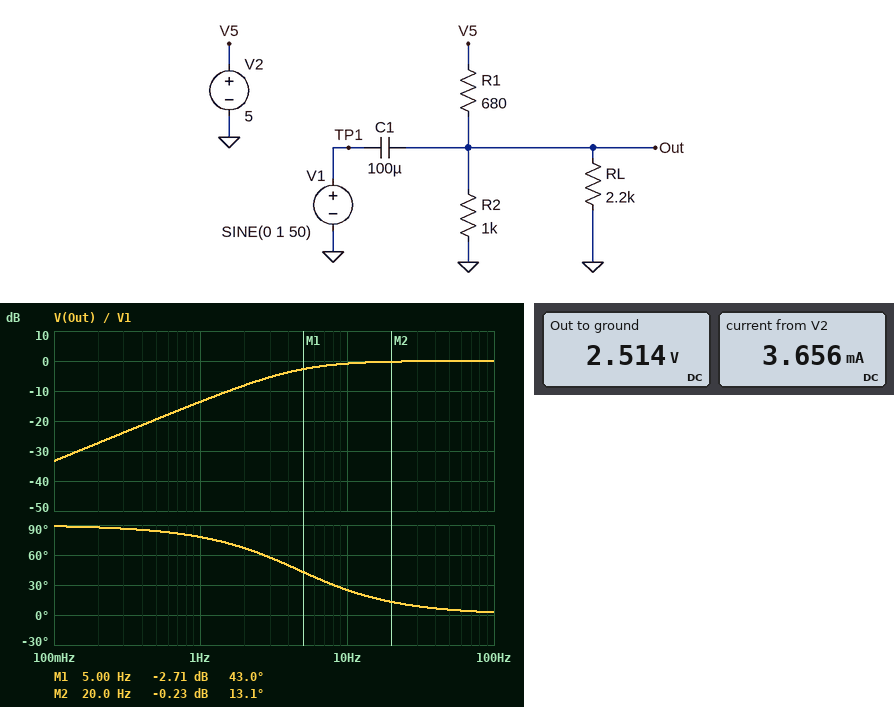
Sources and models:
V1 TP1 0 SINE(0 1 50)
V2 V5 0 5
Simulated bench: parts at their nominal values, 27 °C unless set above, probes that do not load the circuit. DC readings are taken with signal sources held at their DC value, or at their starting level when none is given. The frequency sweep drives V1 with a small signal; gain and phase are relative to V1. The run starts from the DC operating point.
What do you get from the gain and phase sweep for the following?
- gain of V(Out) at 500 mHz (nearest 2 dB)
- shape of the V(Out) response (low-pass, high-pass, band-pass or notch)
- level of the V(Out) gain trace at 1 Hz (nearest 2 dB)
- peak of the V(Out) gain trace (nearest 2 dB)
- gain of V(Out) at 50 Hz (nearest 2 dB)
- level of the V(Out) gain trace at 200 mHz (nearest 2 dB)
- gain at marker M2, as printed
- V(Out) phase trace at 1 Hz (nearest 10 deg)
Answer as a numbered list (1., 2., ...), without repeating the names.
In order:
1. -20 dB
2. high-pass
3. -14 dB
4. 0 dB
5. 0 dB
6. -28 dB
7. -0.23 dB
8. 80 deg
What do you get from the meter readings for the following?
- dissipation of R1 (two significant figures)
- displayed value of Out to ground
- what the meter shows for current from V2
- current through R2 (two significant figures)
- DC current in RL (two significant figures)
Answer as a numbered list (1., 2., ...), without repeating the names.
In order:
1. 9.1 mW
2. 2.514 V
3. 3.656 mA
4. 2.5 mA
5. 1.1 mA
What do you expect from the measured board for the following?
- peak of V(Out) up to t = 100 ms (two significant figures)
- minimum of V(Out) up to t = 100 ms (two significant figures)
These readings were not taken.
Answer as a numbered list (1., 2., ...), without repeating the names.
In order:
1. 3.5 V
2. 1.5 V
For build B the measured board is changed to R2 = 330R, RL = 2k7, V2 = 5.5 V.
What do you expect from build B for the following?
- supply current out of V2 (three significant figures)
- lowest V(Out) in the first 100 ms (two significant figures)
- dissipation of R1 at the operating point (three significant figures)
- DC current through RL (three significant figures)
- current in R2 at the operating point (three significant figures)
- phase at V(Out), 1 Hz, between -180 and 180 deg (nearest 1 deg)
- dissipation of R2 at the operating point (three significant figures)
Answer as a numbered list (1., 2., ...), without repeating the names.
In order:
1. 5.65 mA
2. 600 mV
3. 21.7 mW
4. 615 µA
5. 5.03 mA
6. 83 deg
7. 8.35 mW
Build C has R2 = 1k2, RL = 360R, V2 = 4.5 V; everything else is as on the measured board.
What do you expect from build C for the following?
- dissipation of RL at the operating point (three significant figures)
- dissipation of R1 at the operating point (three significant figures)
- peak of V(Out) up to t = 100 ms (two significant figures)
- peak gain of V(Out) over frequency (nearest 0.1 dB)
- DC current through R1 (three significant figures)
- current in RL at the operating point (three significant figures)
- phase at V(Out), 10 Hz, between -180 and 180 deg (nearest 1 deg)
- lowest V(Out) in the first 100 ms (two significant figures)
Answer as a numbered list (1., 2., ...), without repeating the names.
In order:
1. 4.71 mW
2. 15.0 mW
3. 2.3 V
4. 0 dB
5. 4.70 mA
6. 3.62 mA
7. 39 deg
8. 240 mV
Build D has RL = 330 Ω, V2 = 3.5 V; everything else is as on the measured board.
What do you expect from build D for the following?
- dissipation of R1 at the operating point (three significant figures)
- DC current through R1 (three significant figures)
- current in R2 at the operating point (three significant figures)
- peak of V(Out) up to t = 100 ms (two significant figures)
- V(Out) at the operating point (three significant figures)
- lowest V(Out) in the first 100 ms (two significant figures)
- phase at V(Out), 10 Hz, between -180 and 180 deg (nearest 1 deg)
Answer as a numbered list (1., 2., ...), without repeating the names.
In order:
1. 9.67 mW
2. 3.77 mA
3. 936 µA
4. 1.9 V
5. 936 mV
6. -130 mV
7. 41 deg
